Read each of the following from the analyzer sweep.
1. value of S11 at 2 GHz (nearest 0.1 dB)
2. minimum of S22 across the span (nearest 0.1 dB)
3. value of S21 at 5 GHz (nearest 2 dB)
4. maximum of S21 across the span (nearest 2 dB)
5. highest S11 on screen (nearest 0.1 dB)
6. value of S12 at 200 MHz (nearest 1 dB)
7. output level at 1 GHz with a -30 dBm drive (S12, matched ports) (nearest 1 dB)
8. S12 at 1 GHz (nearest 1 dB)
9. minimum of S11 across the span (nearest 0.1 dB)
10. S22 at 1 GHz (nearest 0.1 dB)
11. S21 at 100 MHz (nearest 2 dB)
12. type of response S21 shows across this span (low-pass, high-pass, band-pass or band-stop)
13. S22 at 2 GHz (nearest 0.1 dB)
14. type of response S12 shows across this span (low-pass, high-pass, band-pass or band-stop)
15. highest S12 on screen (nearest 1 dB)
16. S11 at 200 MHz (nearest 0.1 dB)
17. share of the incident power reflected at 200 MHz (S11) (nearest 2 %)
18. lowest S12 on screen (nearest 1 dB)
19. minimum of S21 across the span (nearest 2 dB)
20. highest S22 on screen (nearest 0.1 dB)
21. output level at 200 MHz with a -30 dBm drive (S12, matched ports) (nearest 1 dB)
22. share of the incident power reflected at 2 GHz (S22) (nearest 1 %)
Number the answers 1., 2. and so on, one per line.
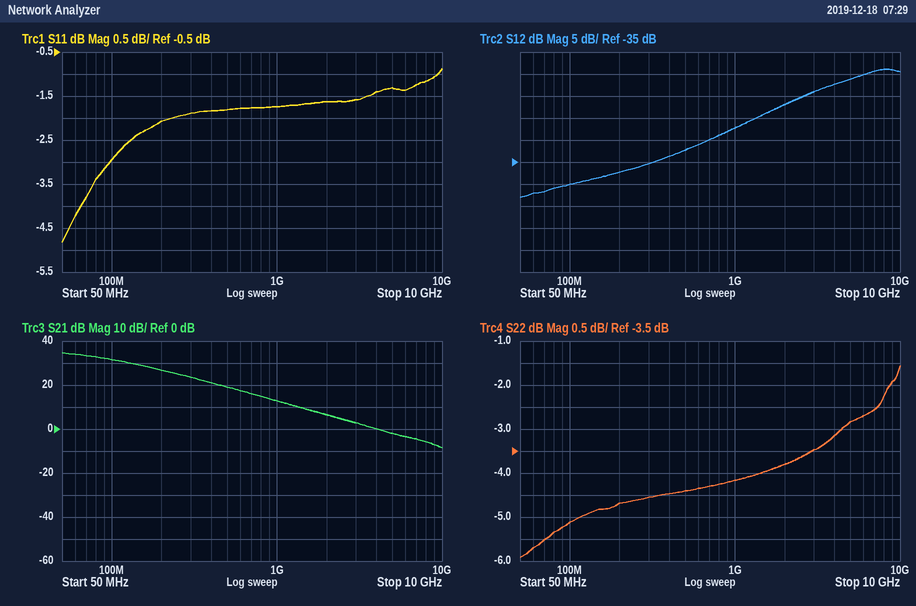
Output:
1. -1.6 dB
2. -5.9 dB
3. -2 dB
4. 34 dB
5. -0.9 dB
6. -37 dB
7. -57 dBm
8. -27 dB
9. -4.8 dB
10. -4.2 dB
11. 32 dB
12. low-pass
13. -3.8 dB
14. high-pass
15. -14 dB
16. -2.1 dB
17. 62 %
18. -43 dB
19. -8 dB
20. -1.6 dB
21. -67 dBm
22. 42 %
